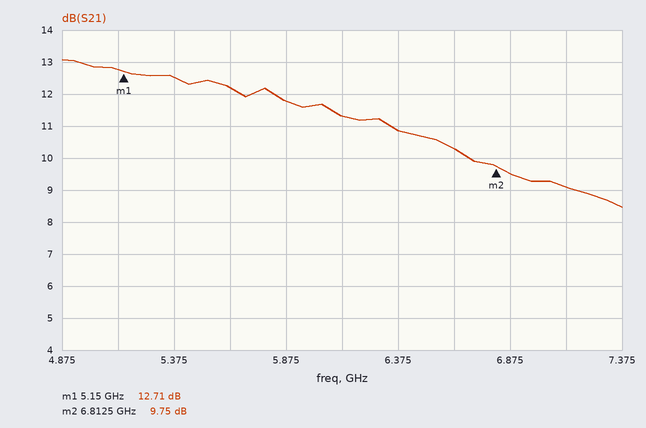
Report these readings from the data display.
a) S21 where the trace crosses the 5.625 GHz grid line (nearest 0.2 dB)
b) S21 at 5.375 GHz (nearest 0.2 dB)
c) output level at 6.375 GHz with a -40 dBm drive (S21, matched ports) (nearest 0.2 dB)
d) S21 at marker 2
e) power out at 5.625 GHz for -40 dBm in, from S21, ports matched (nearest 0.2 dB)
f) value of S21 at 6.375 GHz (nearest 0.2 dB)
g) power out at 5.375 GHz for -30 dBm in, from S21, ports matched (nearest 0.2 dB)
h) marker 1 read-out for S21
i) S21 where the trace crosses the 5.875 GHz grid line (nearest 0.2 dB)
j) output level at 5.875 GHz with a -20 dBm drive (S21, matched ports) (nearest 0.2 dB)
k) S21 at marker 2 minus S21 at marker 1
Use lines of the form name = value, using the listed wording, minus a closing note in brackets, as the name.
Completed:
S21 where the trace crosses the 5.625 GHz grid line = 12.2 dB
S21 at 5.375 GHz = 12.6 dB
output level at 6.375 GHz with a -40 dBm drive (S21, matched ports) = -29.2 dBm
S21 at marker 2 = 9.75 dB
power out at 5.625 GHz for -40 dBm in, from S21, ports matched = -27.8 dBm
value of S21 at 6.375 GHz = 10.8 dB
power out at 5.375 GHz for -30 dBm in, from S21, ports matched = -17.4 dBm
marker 1 read-out for S21 = 12.71 dB
S21 where the trace crosses the 5.875 GHz grid line = 11.8 dB
output level at 5.875 GHz with a -20 dBm drive (S21, matched ports) = -8.2 dBm
S21 at marker 2 minus S21 at marker 1 = -2.96 dB
